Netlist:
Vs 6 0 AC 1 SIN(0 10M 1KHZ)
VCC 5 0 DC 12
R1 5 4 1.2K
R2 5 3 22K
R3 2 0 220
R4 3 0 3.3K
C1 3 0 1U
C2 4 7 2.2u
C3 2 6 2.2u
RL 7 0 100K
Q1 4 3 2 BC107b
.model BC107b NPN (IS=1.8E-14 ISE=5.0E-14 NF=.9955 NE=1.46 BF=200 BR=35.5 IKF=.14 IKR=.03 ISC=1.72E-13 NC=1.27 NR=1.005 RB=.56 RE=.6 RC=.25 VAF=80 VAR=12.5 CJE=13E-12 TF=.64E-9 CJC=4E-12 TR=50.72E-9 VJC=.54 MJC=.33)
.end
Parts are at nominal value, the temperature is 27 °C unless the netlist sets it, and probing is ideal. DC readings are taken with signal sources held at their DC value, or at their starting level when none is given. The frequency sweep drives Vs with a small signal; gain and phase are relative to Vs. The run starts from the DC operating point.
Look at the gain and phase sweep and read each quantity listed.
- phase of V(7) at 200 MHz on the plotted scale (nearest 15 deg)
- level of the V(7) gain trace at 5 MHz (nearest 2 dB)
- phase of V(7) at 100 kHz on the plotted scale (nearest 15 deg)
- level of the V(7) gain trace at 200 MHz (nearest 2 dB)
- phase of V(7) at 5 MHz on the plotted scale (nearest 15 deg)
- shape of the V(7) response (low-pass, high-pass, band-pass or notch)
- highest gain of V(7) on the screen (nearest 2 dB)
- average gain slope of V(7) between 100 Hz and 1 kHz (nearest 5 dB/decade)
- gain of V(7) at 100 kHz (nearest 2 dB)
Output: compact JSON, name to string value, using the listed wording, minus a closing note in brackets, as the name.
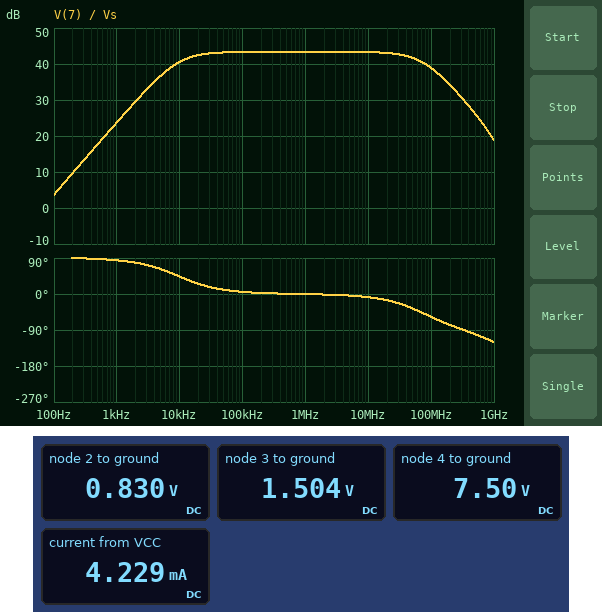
{"phase of V(7) at 200 MHz on the plotted scale": "-75 deg", "level of the V(7) gain trace at 5 MHz": "44 dB", "phase of V(7) at 100 kHz on the plotted scale": "0 deg", "level of the V(7) gain trace at 200 MHz": "34 dB", "phase of V(7) at 5 MHz on the plotted scale": "0 deg", "shape of the V(7) response": "band-pass", "highest gain of V(7) on the screen": "44 dB", "average gain slope of V(7) between 100 Hz and 1 kHz": "20 dB/decade", "gain of V(7) at 100 kHz": "44 dB"}
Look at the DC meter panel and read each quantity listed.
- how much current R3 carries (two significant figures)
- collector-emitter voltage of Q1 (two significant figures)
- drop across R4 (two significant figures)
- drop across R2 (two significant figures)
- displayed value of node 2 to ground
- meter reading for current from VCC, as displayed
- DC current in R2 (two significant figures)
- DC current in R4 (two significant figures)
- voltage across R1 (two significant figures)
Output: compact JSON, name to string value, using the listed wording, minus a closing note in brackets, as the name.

{"how much current R3 carries": "3.8 mA", "collector-emitter voltage of Q1": "6.7 V", "drop across R4": "1.5 V", "drop across R2": "10 V", "displayed value of node 2 to ground": "0.830 V", "meter reading for current from VCC, as displayed": "4.229 mA", "DC current in R2": "480 µA", "DC current in R4": "460 µA", "voltage across R1": "4.5 V"}
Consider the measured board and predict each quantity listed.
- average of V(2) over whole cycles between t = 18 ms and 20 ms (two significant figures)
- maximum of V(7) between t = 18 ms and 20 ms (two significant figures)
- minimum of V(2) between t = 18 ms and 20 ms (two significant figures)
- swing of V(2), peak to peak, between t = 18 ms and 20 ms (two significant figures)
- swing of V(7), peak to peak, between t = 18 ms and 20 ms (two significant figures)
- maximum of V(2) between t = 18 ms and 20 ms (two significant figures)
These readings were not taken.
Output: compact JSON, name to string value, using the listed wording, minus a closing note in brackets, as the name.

{"average of V(2) over whole cycles between t = 18 ms and 20 ms": "830 mV", "maximum of V(7) between t = 18 ms and 20 ms": "150 mV", "minimum of V(2) between t = 18 ms and 20 ms": "830 mV", "swing of V(2), peak to peak, between t = 18 ms and 20 ms": "2.1 mV", "swing of V(7), peak to peak, between t = 18 ms and 20 ms": "310 mV", "maximum of V(2) between t = 18 ms and 20 ms": "830 mV"}
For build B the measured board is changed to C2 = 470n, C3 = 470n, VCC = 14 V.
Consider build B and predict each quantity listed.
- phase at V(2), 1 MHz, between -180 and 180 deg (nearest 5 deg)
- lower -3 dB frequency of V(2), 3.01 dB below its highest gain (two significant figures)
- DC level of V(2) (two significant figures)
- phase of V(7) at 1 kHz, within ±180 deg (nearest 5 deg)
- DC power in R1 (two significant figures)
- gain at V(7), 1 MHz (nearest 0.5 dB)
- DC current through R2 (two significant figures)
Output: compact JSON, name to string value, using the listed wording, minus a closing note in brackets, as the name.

{"phase at V(2), 1 MHz, between -180 and 180 deg": "5 deg", "lower -3 dB frequency of V(2), 3.01 dB below its highest gain": "54 kHz", "DC level of V(2)": "1.1 V", "phase of V(7) at 1 kHz, within ±180 deg": "90 deg", "DC power in R1": "28 mW", "gain at V(7), 1 MHz": "45.0 dB", "DC current through R2": "560 µA"}
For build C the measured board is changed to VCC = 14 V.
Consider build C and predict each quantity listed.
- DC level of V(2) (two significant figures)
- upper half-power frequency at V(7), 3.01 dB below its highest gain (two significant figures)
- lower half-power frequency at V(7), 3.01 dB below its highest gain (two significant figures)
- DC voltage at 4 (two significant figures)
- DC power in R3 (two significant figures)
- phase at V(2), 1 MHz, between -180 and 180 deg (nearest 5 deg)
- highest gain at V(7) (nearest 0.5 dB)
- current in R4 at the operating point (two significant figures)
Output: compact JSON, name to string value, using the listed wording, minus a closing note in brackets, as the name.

{"DC level of V(2)": "1.1 V", "upper half-power frequency at V(7), 3.01 dB below its highest gain": "76 MHz", "lower half-power frequency at V(7), 3.01 dB below its highest gain": "12 kHz", "DC voltage at 4": "8.2 V", "DC power in R3": "5.2 mW", "phase at V(2), 1 MHz, between -180 and 180 deg": "0 deg", "highest gain at V(7)": "45.0 dB", "current in R4 at the operating point": "530 µA"}
